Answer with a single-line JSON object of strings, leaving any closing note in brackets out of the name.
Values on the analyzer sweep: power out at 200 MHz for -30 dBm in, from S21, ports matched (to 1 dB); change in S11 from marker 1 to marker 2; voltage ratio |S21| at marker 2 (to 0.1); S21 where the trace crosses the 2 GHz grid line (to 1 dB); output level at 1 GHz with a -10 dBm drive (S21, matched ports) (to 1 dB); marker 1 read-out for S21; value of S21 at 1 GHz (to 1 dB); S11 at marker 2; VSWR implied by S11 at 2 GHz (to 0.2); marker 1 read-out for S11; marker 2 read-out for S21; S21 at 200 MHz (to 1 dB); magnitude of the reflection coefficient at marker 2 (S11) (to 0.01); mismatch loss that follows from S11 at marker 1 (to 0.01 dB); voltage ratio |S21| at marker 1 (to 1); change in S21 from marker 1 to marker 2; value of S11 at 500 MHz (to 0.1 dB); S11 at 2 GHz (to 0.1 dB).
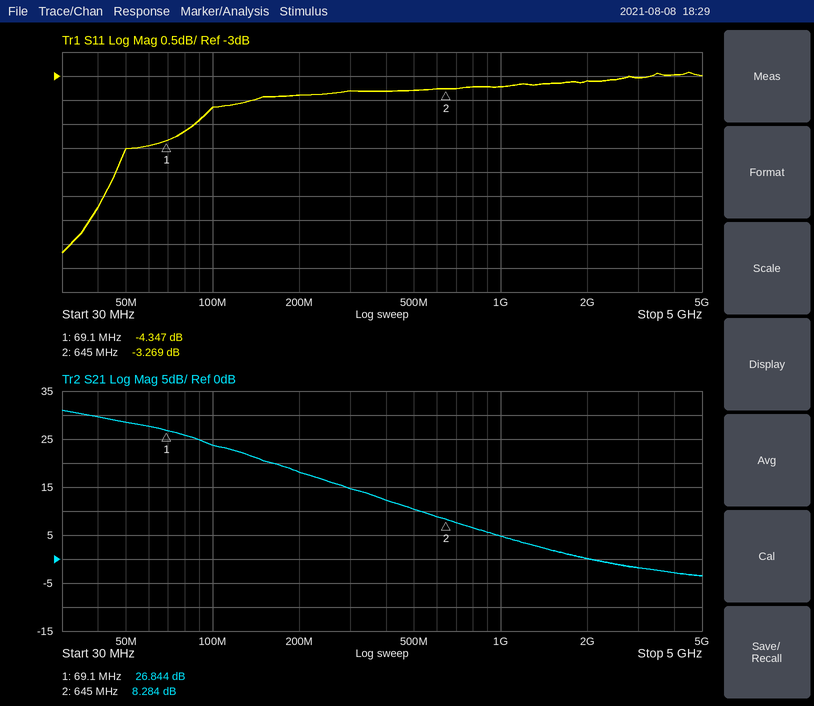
{"power out at 200 MHz for -30 dBm in, from S21, ports matched": "-12 dBm", "change in S11 from marker 1 to marker 2": "1.078 dB", "voltage ratio |S21| at marker 2": "2.6", "S21 where the trace crosses the 2 GHz grid line": "0 dB", "output level at 1 GHz with a -10 dBm drive (S21, matched ports)": "-5 dBm", "marker 1 read-out for S21": "26.844 dB", "value of S21 at 1 GHz": "5 dB", "S11 at marker 2": "-3.269 dB", "VSWR implied by S11 at 2 GHz": "5.6", "marker 1 read-out for S11": "-4.347 dB", "marker 2 read-out for S21": "8.284 dB", "S21 at 200 MHz": "18 dB", "magnitude of the reflection coefficient at marker 2 (S11)": "0.69", "mismatch loss that follows from S11 at marker 1": "1.99 dB", "voltage ratio |S21| at marker 1": "22", "change in S21 from marker 1 to marker 2": "-18.560 dB", "value of S11 at 500 MHz": "-3.3 dB", "S11 at 2 GHz": "-3.1 dB"}
